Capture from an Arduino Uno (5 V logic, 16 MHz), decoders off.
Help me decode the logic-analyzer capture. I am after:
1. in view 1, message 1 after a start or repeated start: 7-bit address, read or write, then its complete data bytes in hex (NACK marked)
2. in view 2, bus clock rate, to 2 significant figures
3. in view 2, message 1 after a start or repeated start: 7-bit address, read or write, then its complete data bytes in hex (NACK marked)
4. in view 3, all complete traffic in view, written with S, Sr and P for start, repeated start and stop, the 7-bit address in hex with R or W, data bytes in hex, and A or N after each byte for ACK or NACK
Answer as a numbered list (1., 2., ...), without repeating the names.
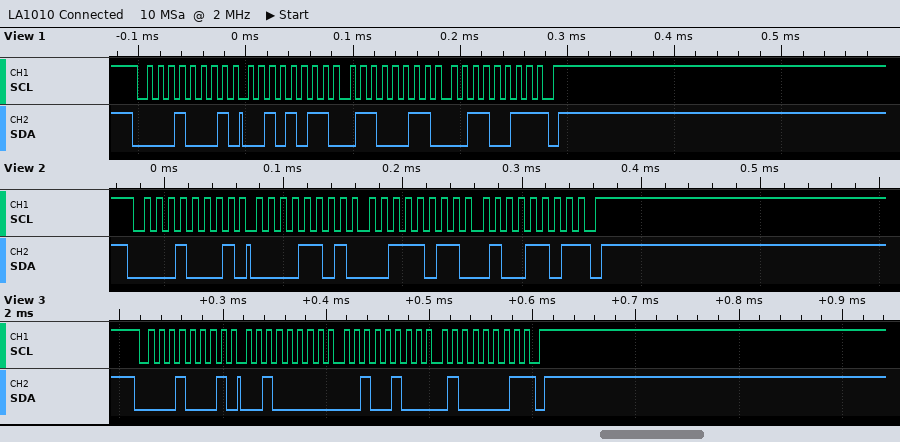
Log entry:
1. 0x08 read: 2B 63 33 NACK
2. 100 kHz
3. 0x08 read: 0D 3B 4D NACK
4. S 08R A 20 A 24 A 41 N P
